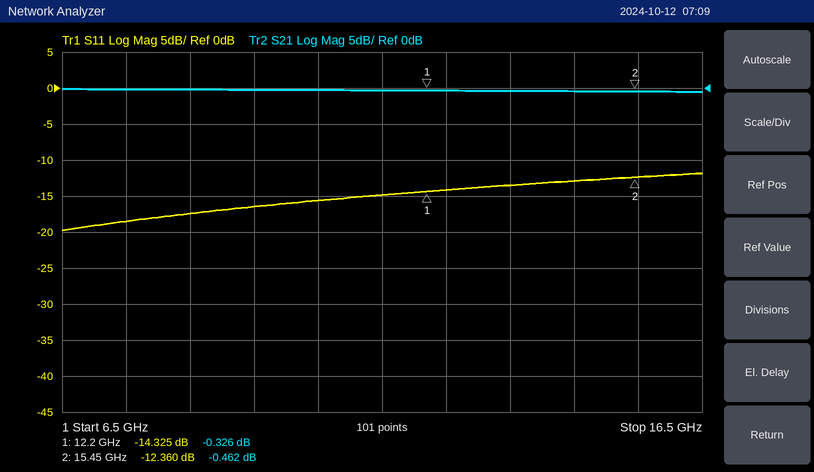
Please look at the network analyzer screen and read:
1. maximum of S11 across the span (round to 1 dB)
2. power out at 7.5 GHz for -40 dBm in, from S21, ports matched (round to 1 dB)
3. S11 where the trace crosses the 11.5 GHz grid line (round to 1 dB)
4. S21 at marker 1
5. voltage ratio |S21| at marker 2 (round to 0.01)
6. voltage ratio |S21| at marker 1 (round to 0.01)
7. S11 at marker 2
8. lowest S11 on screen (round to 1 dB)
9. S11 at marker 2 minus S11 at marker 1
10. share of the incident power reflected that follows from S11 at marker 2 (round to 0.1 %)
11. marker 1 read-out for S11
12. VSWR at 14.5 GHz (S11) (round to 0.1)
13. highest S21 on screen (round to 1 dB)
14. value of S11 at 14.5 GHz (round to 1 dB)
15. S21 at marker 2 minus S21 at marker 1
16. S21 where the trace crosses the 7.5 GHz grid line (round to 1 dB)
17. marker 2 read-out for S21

-12 dB
-40 dBm
-15 dB
-0.326 dB
0.95
0.96
-12.360 dB
-20 dB
1.965 dB
5.8 %
-14.325 dB
1.6
0 dB
-13 dB
-0.136 dB
0 dB
-0.462 dB
